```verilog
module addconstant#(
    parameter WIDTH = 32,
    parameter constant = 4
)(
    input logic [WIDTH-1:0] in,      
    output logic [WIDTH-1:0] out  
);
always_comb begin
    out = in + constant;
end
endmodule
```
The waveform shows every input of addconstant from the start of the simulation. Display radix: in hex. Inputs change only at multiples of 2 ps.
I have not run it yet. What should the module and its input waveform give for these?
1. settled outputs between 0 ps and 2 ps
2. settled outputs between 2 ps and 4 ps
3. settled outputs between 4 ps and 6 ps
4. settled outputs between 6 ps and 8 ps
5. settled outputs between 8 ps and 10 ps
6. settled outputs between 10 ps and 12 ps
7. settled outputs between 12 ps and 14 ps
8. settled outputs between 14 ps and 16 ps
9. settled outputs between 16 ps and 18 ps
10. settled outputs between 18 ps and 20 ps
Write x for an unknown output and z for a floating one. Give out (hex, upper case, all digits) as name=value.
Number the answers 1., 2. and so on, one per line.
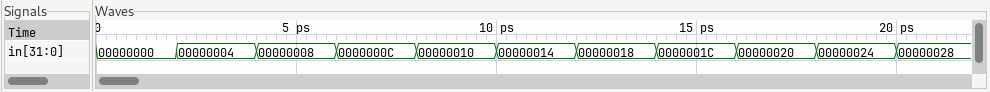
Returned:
1. out=00000004
2. out=00000008
3. out=0000000C
4. out=00000010
5. out=00000014
6. out=00000018
7. out=0000001C
8. out=00000020
9. out=00000024
10. out=00000028
